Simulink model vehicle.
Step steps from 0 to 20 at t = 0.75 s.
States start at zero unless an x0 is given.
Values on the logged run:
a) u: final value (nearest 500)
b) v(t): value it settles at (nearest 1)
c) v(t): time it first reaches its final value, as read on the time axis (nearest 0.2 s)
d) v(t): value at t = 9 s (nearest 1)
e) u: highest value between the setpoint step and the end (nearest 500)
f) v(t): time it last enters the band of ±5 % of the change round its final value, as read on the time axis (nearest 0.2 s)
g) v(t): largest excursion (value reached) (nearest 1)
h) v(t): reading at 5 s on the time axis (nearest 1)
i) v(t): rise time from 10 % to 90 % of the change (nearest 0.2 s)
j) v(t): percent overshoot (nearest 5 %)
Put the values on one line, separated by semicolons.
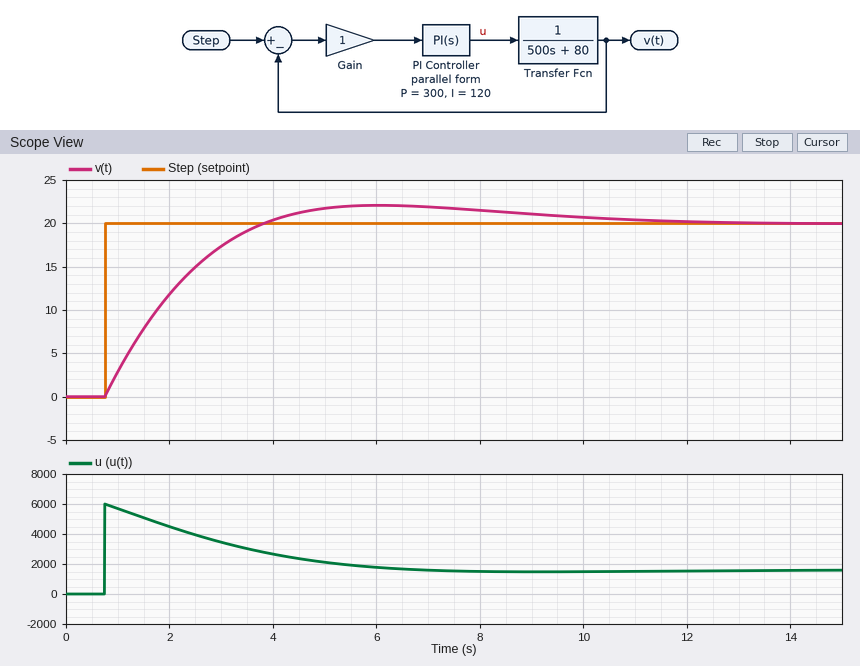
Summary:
1500; 20; 3.8 s; 21; 6000; 9.2 s; 22; 22; 2.2 s; 10 %
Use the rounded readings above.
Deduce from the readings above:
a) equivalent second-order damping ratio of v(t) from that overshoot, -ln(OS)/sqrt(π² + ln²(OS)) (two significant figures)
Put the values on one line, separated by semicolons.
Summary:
0.59
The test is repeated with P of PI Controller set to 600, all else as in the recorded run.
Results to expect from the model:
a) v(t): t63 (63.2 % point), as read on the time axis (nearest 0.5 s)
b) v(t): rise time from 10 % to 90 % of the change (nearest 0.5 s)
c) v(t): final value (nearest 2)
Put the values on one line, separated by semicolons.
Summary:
1.5 s; 1.5 s; 20
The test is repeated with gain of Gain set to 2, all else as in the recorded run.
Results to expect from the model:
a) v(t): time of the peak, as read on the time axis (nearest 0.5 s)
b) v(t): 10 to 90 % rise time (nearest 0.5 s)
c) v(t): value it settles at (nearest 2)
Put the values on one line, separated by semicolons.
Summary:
4.0 s; 1.5 s; 20
